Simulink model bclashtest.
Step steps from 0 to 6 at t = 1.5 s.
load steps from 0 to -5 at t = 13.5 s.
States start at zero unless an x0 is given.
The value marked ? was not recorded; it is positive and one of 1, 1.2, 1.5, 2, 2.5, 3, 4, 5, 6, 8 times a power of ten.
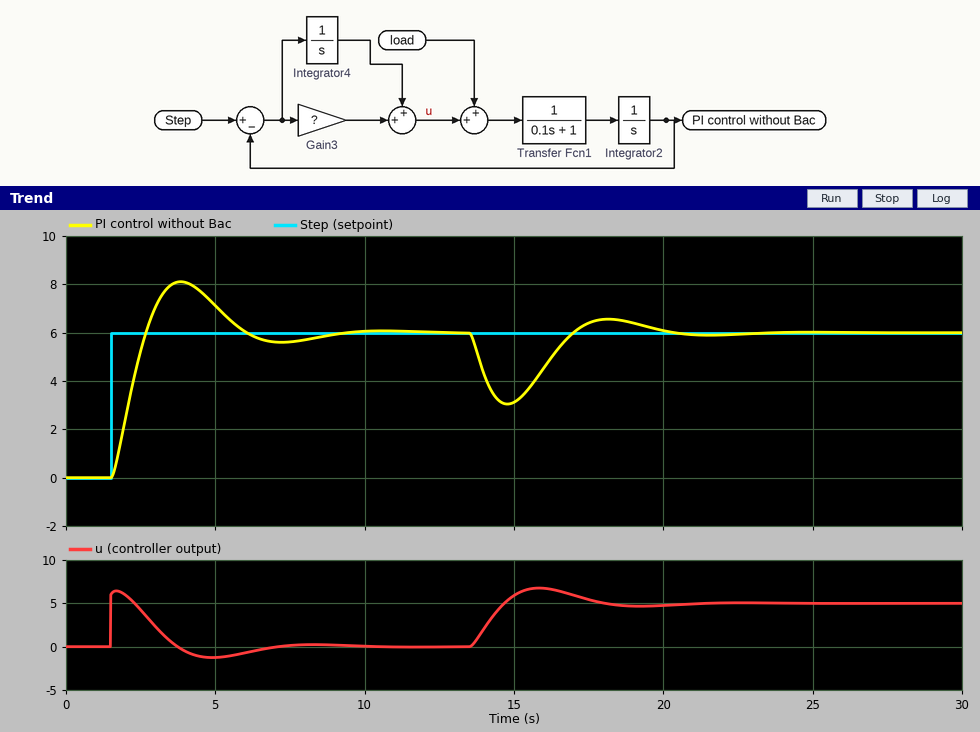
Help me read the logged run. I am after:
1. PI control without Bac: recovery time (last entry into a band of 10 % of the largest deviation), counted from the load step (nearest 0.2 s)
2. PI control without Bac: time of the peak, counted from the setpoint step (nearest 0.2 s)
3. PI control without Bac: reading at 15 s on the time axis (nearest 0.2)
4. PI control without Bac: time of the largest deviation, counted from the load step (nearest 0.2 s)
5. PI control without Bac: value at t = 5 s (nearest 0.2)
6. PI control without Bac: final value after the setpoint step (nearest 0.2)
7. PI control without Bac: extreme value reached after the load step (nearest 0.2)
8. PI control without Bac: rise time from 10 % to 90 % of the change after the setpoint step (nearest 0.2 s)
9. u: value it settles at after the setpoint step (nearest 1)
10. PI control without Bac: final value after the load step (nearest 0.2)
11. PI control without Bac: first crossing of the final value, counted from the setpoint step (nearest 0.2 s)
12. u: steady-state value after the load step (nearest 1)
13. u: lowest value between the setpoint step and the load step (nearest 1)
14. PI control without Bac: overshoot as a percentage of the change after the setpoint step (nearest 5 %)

5.8 s
2.4 s
3.2
1.2 s
7.2
6.0
3.0
0.8 s
0
6.0
1.2 s
5
-1
35 %
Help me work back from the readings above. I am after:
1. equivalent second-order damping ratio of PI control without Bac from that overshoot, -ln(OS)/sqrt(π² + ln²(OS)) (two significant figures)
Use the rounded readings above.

0.32
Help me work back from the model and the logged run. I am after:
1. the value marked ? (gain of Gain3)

1
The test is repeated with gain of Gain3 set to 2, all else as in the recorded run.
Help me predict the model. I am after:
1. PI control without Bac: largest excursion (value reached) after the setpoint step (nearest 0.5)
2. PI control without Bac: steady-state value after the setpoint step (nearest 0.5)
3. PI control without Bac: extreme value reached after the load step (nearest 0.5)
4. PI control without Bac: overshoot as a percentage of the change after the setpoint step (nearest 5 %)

7.0
6.0
4.0
15 %
